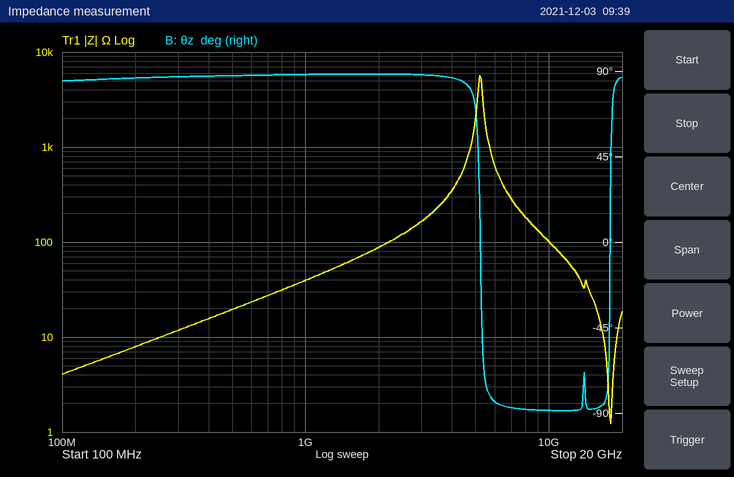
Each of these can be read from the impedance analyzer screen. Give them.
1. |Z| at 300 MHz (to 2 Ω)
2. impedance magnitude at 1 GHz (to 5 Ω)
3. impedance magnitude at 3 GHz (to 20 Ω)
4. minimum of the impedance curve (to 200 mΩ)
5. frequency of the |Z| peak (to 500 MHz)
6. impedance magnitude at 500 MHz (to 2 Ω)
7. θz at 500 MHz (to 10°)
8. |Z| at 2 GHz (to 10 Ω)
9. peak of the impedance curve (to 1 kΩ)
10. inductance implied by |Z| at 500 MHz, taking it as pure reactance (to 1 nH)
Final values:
12 Ω
40 Ω
160 Ω
1.2 Ω
5.0 GHz
20 Ω
90°
90 Ω
6 kΩ
6 nH
